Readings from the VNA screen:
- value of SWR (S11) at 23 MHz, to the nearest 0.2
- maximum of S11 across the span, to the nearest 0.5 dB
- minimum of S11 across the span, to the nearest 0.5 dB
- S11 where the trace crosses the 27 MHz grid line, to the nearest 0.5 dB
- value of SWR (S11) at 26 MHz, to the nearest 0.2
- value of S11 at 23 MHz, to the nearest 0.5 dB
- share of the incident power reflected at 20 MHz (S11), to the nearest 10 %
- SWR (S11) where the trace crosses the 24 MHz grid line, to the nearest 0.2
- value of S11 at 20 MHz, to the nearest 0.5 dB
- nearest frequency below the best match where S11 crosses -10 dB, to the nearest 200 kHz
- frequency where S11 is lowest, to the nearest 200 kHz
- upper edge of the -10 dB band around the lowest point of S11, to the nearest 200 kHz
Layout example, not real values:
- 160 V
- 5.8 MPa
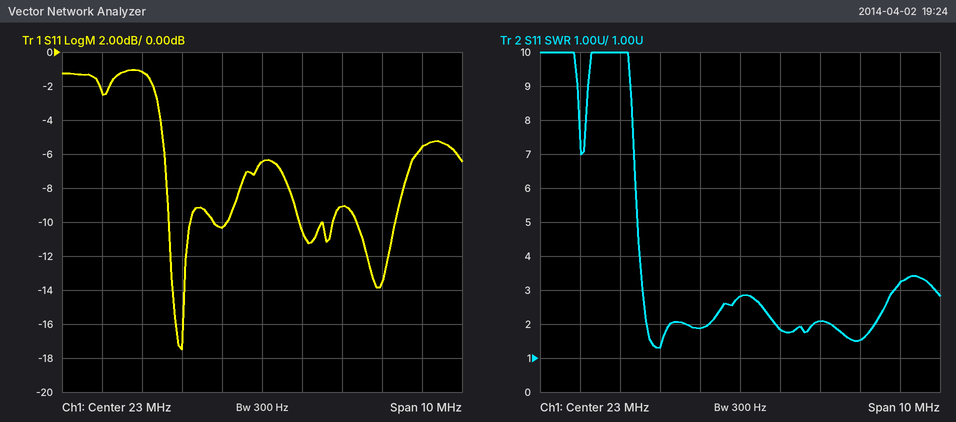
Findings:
- 2.8
- -1.0 dB
- -17.5 dB
- -5.5 dB
- 1.6
- -6.5 dB
- 80 %
- 1.8
- -1.0 dB
- 20.6 MHz
- 21.0 MHz
- 21.2 MHz
